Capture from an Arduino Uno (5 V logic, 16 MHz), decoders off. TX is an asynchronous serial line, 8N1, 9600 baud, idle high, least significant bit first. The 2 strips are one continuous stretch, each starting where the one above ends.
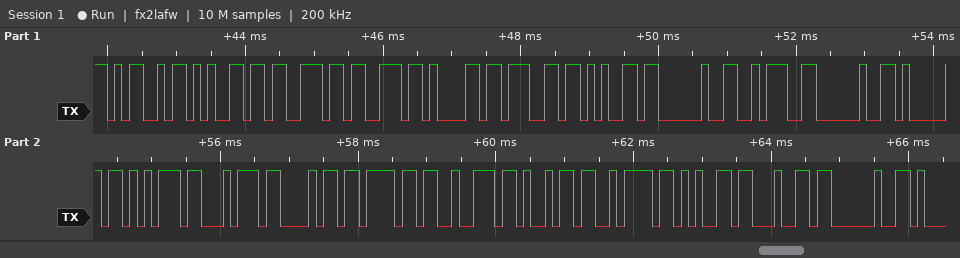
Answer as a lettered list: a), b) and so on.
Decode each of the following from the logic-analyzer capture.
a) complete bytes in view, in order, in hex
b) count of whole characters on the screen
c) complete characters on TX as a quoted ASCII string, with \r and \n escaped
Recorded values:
a) 4D 65 73 73 61 67 65 20 3A 20 41 75 74 68 6F 72 69 7A 65 64 20
b) 21
c) "Message : Authorized "
